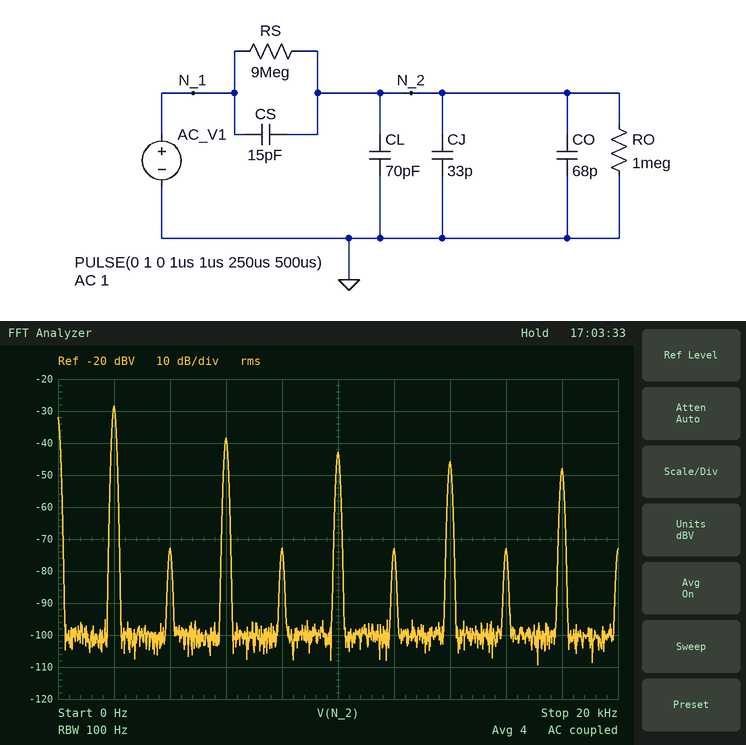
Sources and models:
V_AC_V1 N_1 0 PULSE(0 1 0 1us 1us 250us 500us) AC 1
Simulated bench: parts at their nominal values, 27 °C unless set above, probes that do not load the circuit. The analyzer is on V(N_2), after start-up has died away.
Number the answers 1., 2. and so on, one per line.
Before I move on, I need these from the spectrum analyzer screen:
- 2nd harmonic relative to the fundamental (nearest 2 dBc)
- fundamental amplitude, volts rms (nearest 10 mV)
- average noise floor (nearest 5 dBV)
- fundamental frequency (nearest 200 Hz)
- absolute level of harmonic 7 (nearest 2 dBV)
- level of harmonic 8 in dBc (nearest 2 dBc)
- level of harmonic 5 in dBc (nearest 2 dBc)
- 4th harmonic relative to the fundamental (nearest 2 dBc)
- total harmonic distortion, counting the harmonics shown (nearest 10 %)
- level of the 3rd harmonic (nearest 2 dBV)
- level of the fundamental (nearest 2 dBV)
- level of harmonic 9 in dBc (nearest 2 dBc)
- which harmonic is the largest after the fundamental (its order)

1. -44 dBc
2. 40 mV
3. -100 dBV
4. 2.0 kHz
5. -46 dBV
6. -44 dBc
7. -14 dBc
8. -44 dBc
9. 40 %
10. -38 dBV
11. -28 dBV
12. -20 dBc
13. 3
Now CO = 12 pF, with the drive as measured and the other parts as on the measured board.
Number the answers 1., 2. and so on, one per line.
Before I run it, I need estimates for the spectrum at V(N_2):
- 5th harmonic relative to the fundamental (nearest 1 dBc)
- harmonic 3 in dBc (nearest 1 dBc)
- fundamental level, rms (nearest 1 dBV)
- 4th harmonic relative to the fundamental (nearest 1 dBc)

1. -14 dBc
2. -9 dBc
3. -26 dBV
4. -44 dBc
